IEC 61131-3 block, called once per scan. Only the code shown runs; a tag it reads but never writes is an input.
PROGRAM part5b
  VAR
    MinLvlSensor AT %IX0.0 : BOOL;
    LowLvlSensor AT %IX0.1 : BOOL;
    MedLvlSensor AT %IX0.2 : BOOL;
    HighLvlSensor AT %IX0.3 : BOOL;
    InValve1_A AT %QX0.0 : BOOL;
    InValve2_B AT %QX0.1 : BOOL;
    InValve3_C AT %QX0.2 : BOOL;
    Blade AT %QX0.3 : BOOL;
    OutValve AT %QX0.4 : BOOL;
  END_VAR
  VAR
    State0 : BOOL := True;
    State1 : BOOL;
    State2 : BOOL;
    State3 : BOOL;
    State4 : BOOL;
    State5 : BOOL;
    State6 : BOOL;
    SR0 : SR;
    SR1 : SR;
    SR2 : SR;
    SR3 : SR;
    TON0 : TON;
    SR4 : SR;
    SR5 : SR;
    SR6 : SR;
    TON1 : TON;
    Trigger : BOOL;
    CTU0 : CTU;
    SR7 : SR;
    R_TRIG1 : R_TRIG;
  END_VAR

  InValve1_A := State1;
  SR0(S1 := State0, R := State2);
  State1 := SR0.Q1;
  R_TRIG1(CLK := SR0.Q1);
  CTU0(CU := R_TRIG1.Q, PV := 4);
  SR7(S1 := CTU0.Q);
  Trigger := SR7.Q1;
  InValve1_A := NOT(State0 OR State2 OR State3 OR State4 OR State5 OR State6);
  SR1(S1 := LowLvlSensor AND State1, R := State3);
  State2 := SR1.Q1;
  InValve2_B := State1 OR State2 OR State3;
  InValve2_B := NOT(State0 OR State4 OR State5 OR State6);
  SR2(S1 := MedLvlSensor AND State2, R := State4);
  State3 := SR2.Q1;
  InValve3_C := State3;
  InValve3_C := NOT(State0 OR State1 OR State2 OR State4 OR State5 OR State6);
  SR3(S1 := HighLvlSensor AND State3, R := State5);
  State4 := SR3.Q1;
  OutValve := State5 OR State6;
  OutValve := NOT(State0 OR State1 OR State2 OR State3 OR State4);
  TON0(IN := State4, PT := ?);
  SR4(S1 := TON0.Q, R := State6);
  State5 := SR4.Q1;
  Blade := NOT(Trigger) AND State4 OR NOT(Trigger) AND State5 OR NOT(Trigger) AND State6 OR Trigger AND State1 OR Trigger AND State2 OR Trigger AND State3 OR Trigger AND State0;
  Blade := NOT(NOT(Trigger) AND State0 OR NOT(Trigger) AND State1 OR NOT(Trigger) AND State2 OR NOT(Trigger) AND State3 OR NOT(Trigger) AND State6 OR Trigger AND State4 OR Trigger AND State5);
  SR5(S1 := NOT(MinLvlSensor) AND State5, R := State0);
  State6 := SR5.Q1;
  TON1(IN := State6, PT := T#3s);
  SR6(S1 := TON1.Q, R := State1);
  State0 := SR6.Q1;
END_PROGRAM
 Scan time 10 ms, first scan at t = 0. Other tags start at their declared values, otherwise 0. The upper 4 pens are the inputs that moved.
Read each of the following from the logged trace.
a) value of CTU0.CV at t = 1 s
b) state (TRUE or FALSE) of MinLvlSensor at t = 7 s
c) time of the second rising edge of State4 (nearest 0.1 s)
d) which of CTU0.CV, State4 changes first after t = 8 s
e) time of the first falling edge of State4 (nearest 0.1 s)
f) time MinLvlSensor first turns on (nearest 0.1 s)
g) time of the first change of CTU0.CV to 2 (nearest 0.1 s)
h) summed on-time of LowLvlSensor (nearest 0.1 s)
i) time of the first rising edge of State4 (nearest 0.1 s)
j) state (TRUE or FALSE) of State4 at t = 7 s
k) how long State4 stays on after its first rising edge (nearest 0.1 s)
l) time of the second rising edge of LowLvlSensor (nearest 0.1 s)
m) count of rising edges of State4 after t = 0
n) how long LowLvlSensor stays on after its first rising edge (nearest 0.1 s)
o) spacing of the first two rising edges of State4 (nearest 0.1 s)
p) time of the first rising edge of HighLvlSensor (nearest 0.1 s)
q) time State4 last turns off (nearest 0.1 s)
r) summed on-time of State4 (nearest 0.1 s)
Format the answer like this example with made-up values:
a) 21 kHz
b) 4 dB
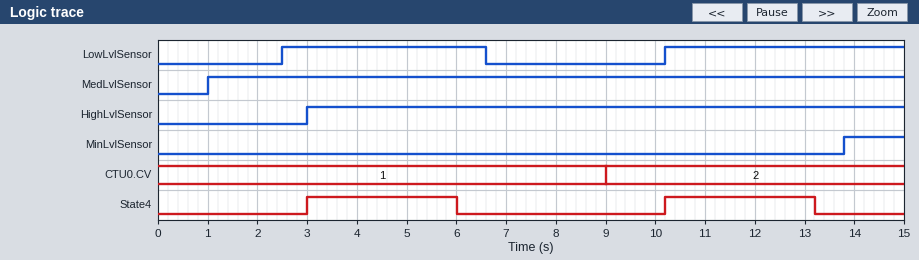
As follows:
a) 1
b) FALSE
c) 10.2 s
d) CTU0.CV
e) 6.0 s
f) 13.8 s
g) 9.0 s
h) 8.9 s
i) 3.0 s
j) FALSE
k) 3.0 s
l) 10.2 s
m) 2
n) 4.1 s
o) 7.2 s
p) 3.0 s
q) 13.2 s
r) 6.0 s
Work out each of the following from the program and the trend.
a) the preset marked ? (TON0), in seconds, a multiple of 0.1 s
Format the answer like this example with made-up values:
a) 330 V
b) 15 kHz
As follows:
a) 3.0 s
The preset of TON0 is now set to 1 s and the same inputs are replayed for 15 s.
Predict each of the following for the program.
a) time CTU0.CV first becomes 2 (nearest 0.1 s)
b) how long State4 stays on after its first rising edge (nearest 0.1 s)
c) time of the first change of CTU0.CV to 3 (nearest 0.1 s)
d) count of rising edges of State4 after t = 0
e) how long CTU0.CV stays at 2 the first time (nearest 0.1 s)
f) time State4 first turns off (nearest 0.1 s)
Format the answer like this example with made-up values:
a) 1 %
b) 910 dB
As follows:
a) 7.0 s
b) 1.0 s
c) 14.2 s
d) 3
e) 7.2 s
f) 4.0 s
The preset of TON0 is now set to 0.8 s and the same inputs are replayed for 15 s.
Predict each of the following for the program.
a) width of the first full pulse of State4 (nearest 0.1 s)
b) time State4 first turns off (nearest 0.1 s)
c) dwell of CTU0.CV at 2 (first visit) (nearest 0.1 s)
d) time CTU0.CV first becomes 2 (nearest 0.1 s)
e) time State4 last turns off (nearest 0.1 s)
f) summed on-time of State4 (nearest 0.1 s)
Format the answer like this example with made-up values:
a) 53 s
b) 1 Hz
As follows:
a) 0.8 s
b) 3.8 s
c) 7.2 s
d) 6.8 s
e) 14.8 s
f) 2.4 s
